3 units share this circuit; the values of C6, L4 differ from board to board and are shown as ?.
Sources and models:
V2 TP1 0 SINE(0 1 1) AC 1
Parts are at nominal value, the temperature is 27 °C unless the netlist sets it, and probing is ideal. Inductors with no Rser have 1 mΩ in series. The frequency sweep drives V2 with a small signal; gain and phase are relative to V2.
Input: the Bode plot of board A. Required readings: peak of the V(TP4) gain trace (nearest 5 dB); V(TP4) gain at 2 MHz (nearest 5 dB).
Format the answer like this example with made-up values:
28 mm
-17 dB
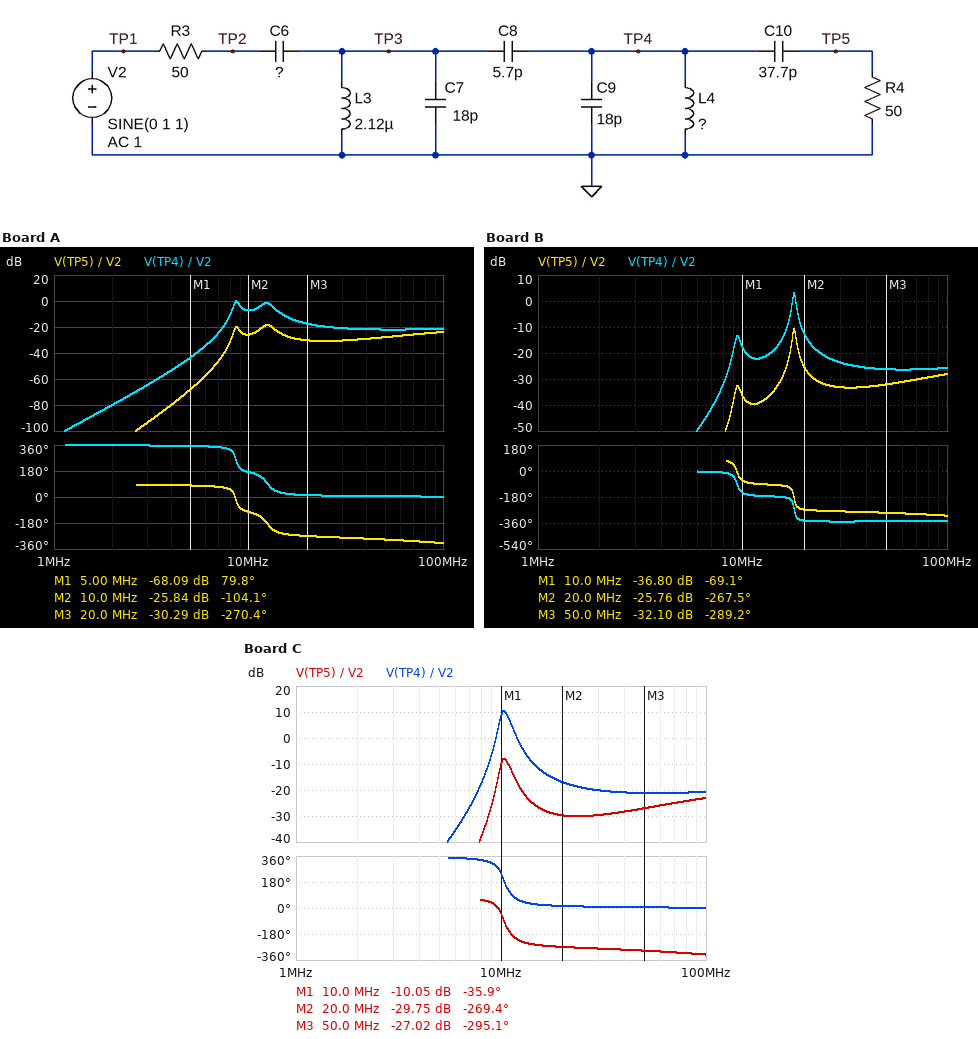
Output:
0 dB
-80 dB
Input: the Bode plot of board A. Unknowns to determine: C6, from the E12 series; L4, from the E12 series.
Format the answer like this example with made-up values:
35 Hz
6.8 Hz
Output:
56 pF
5.6 µH
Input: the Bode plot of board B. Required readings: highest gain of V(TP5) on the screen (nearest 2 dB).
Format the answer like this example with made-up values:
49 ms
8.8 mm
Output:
-10 dB
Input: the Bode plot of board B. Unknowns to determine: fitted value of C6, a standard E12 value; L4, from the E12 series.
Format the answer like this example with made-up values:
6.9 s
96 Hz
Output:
15 pF
4.7 µH
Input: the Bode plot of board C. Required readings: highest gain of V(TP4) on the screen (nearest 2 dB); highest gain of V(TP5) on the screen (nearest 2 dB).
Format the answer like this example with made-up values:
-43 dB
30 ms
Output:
10 dB
-8 dB
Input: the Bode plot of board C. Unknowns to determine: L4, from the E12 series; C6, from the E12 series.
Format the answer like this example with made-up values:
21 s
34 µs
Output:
3.9 µH
82 pF
